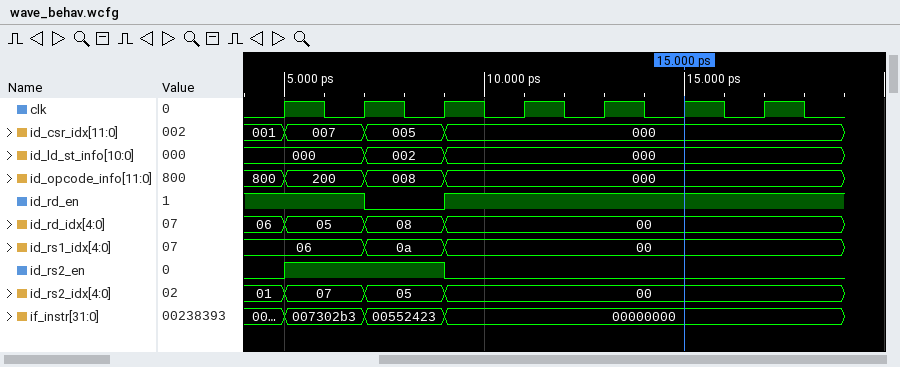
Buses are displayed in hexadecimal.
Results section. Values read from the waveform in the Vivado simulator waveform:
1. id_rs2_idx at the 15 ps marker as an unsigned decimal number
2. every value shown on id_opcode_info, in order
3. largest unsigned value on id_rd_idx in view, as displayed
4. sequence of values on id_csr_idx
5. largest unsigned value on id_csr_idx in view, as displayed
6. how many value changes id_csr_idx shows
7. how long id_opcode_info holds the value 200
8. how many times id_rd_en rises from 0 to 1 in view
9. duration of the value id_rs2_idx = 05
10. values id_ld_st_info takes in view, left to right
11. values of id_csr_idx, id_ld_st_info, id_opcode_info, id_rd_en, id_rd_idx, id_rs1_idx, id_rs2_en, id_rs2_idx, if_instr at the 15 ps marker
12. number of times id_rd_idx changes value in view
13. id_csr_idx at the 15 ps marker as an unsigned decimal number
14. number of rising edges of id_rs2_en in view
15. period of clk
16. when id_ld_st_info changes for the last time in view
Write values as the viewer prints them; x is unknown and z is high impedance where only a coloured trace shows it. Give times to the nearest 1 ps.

0
800, 200, 008, 000
08
001, 007, 005, 000
007
3
2 ps
1
2 ps
000, 002, 000
id_csr_idx=000, id_ld_st_info=000, id_opcode_info=000, id_rd_en=1, id_rd_idx=00, id_rs1_idx=00, id_rs2_en=0, id_rs2_idx=00, if_instr=00000000
3
0
1
2 ps
9 ps
